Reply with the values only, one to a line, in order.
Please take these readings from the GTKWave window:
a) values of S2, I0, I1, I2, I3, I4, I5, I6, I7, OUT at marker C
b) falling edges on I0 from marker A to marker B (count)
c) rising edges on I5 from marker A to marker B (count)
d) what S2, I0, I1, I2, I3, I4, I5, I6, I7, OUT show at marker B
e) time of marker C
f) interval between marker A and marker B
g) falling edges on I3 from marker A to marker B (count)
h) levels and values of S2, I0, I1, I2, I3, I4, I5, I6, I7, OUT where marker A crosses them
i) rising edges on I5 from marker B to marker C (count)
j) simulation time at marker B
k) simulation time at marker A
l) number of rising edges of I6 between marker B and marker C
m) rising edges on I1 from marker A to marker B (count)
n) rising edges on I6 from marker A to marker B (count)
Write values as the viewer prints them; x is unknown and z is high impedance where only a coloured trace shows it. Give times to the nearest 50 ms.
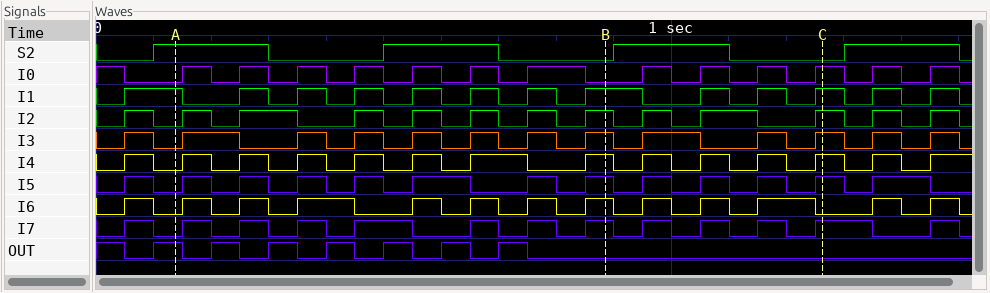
S2=0, I0=1, I1=1, I2=1, I3=1, I4=1, I5=1, I6=0, I7=1, OUT=0
7
7
S2=0, I0=0, I1=1, I2=1, I3=1, I4=1, I5=1, I6=1, I7=1, OUT=0
1250 ms
750 ms
6
S2=1, I0=0, I1=1, I2=0, I3=0, I4=0, I5=0, I6=0, I7=0, OUT=1
4
900 ms
150 ms
3
7
7
